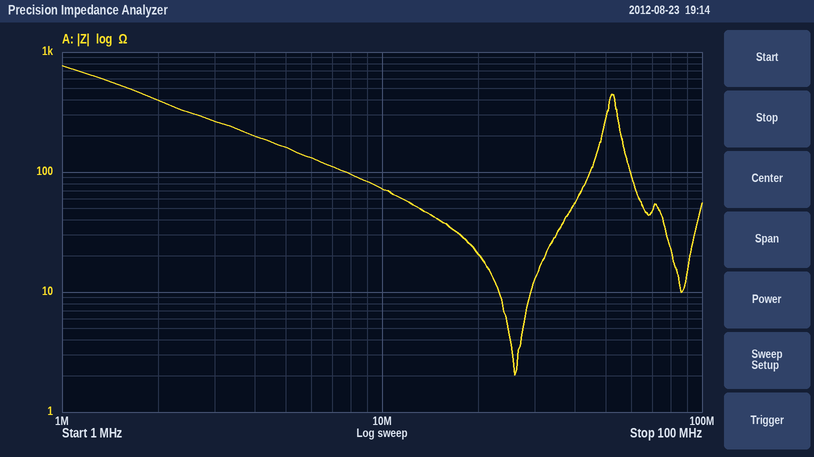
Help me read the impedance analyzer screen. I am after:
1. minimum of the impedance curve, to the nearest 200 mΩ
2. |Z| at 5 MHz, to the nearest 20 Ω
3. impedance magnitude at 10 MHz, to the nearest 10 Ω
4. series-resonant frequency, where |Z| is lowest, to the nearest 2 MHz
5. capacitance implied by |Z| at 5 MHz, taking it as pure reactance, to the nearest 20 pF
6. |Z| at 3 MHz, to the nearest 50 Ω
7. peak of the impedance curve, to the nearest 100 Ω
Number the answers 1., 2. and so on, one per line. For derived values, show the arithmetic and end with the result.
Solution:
1. 2.0 Ω
2. 160 Ω
3. 70 Ω
4. 26 MHz
5. C = 1/(2π × 5 MHz × 160 Ω) ≈ 199 pF, so 200 pF to the nearest 20 pF
6. 250 Ω
7. 800 Ω
